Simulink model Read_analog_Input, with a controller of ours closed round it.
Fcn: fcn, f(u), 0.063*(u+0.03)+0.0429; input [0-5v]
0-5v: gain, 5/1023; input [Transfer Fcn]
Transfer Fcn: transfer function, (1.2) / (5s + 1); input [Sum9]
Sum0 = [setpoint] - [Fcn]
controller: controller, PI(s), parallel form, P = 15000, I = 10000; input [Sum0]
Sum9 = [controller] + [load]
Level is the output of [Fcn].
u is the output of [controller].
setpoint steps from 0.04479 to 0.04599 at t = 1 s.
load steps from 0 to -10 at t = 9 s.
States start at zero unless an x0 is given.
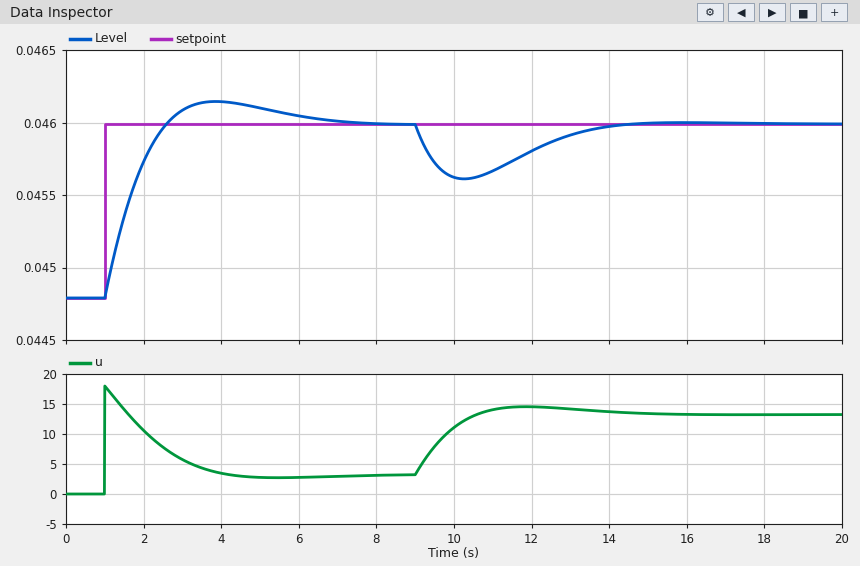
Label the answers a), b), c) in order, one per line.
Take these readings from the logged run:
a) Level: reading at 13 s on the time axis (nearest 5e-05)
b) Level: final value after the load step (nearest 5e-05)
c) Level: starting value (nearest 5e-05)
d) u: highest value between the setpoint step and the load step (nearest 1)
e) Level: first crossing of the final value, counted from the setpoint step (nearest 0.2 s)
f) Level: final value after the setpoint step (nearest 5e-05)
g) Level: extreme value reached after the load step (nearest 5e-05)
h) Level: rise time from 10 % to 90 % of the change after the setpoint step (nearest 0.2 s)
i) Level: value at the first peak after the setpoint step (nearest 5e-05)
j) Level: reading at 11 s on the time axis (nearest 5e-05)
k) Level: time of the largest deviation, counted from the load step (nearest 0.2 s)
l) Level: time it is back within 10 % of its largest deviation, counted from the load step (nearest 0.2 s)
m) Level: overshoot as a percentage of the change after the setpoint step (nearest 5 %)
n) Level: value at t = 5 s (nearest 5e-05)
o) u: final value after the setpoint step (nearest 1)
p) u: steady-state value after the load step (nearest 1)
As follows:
a) 0.04590
b) 0.04600
c) 0.04480
d) 18
e) 1.6 s
f) 0.04600
g) 0.04560
h) 1.2 s
i) 0.04615
j) 0.04565
k) 1.2 s
l) 4.6 s
m) 15 %
n) 0.04610
o) 3
p) 13
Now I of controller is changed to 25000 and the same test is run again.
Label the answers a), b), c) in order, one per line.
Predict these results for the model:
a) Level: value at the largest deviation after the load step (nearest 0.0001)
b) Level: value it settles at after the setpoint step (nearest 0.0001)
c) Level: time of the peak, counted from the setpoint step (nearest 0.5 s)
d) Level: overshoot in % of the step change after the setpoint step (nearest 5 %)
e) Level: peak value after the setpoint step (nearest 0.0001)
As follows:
a) 0.0457
b) 0.0460
c) 2.0 s
d) 25 %
e) 0.0463
